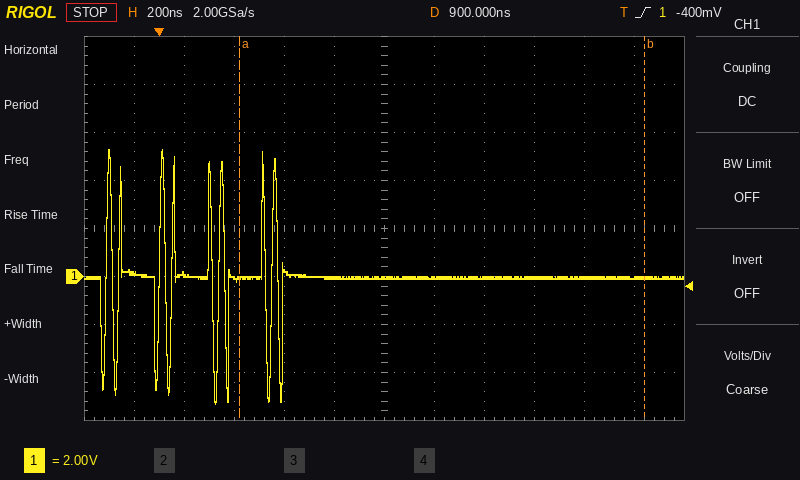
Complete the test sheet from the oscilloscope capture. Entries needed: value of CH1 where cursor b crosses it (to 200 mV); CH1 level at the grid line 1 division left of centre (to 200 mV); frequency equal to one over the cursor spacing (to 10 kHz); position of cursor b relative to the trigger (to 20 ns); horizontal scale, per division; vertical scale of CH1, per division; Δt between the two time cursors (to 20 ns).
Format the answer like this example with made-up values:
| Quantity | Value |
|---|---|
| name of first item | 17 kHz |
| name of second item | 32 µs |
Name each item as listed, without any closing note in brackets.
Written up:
| Quantity | Value |
|---|---|
| value of CH1 where cursor b crosses it | 0.0 V |
| CH1 level at the grid line 1 division left of centre | 0.0 V |
| frequency equal to one over the cursor spacing | 620 kHz |
| position of cursor b relative to the trigger | +1.94 µs |
| horizontal scale, per division | 200 ns |
| vertical scale of CH1, per division | 2 V |
| Δt between the two time cursors | 1.62 µs |
